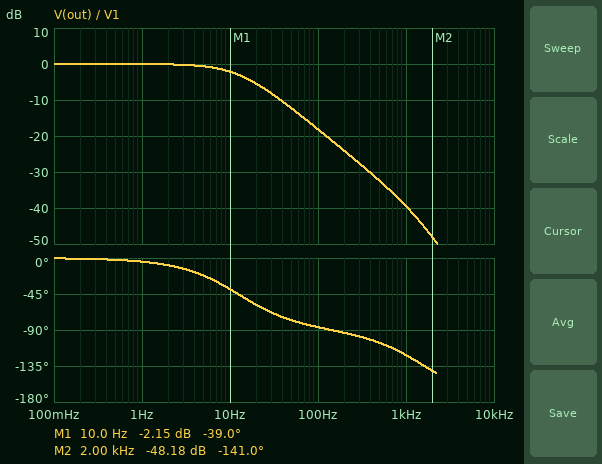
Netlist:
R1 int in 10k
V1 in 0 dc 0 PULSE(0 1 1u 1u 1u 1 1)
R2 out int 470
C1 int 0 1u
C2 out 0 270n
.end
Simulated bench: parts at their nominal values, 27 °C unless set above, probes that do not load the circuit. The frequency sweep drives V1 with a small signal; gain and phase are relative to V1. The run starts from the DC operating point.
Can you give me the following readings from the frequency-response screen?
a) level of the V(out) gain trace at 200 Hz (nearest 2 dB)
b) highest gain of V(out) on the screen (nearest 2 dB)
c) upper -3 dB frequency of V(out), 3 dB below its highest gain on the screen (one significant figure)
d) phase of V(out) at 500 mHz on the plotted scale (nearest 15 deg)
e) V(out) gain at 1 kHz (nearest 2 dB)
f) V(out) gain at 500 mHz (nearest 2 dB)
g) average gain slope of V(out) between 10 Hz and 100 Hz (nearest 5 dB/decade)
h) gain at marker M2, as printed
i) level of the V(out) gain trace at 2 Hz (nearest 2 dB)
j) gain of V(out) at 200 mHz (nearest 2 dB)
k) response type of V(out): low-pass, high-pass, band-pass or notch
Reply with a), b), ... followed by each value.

a) -24 dB
b) 0 dB
c) 10 Hz
d) 0 deg
e) -40 dB
f) 0 dB
g) -15 dB/decade
h) -48.18 dB
i) 0 dB
j) 0 dB
k) low-pass
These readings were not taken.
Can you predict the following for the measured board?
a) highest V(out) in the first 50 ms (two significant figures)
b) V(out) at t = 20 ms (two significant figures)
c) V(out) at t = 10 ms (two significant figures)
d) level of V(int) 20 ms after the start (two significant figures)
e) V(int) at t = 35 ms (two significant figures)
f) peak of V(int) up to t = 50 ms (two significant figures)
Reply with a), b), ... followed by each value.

a) 980 mV
b) 790 mV
c) 540 mV
d) 790 mV
e) 940 mV
f) 980 mV
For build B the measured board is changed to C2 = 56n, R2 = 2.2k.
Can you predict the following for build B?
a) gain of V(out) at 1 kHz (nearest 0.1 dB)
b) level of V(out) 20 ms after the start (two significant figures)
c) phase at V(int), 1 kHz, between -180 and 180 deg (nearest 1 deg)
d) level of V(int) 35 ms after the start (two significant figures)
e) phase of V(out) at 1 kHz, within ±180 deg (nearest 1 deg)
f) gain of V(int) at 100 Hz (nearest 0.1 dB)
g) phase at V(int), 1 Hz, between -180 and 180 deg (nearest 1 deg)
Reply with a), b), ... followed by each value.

a) -38.3 dB
b) 850 mV
c) -88 deg
d) 960 mV
e) -125 deg
f) -16.5 dB
g) -4 deg
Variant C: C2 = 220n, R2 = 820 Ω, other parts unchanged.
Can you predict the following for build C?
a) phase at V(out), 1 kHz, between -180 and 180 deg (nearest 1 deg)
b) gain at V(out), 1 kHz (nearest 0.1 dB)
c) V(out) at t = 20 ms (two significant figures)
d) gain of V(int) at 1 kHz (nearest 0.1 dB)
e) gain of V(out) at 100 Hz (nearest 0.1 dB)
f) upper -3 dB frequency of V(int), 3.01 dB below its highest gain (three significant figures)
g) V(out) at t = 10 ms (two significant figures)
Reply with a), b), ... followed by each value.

a) -132 deg
b) -40.4 dB
c) 800 mV
d) -36.8 dB
e) -17.8 dB
f) 13.0 Hz
g) 550 mV
